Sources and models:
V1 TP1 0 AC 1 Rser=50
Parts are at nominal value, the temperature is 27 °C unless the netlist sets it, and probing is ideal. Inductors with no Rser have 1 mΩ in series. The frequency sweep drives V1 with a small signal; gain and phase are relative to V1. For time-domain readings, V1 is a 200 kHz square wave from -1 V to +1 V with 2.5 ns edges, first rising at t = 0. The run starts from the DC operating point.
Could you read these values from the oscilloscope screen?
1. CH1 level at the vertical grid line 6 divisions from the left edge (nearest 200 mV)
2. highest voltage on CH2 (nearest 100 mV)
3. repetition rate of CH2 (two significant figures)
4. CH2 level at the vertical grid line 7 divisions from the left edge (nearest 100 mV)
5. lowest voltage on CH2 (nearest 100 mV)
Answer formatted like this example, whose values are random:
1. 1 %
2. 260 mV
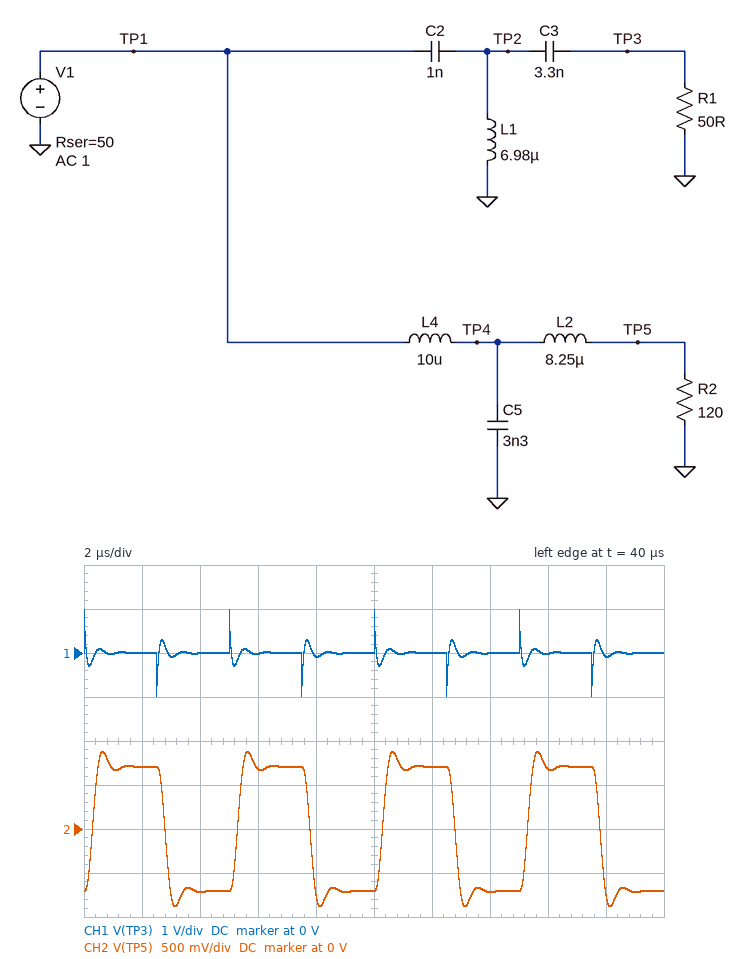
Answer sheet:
1. 0 V
2. 900 mV
3. 200 kHz
4. -700 mV
5. -900 mV
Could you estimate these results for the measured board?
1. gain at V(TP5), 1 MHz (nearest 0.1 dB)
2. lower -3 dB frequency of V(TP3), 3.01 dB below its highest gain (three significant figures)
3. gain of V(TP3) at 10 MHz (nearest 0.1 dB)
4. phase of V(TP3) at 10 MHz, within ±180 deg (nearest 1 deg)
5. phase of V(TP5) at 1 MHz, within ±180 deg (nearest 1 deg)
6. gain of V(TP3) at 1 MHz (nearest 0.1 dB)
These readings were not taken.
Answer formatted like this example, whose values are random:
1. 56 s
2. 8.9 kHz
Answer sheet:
1. -3.3 dB
2. 1.44 MHz
3. -6.1 dB
4. 17 deg
5. -111 deg
6. -18.0 dB
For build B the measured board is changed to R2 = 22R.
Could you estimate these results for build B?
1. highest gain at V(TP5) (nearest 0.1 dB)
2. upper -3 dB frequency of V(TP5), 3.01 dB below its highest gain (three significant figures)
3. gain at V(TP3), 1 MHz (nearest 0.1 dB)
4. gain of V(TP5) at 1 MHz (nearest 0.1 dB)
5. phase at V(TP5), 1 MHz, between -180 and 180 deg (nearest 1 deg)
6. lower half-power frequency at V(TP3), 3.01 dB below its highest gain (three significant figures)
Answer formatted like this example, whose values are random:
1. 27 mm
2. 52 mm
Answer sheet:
1. -10.3 dB
2. 1.45 MHz
3. -13.1 dB
4. -11.2 dB
5. -112 deg
6. 1.55 MHz
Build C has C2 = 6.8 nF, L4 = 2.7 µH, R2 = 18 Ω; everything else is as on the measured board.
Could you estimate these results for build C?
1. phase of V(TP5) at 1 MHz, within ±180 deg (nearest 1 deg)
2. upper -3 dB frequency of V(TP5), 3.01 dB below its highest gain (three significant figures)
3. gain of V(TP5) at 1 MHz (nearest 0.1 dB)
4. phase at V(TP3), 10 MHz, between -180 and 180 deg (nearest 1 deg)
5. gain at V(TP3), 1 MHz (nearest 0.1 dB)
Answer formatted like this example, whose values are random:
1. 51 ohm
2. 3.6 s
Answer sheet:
1. -66 deg
2. 487 kHz
3. -16.5 dB
4. 16 deg
5. -7.6 dB
